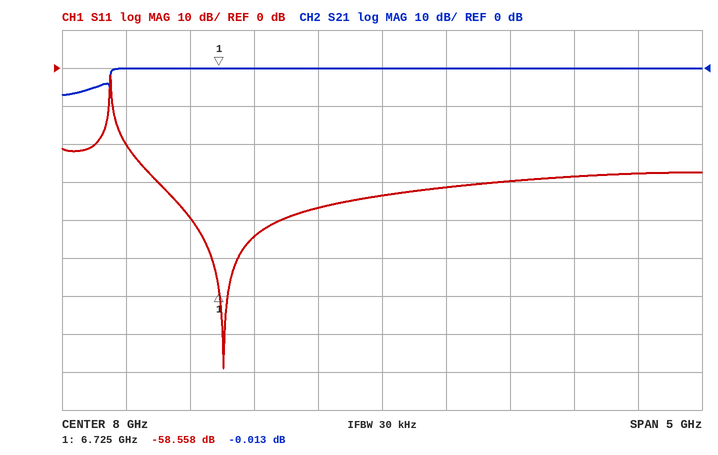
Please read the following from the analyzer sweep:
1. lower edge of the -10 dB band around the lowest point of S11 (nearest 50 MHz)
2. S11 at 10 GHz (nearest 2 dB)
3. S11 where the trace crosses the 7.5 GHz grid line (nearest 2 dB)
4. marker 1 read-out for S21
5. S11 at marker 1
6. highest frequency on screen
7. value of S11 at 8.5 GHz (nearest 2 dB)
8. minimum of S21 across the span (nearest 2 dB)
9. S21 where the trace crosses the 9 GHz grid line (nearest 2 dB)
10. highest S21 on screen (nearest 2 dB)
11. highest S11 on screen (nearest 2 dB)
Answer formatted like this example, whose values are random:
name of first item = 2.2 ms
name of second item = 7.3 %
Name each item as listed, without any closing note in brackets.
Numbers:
lower edge of the -10 dB band around the lowest point of S11 = 5.90 GHz
S11 at 10 GHz = -28 dB
S11 where the trace crosses the 7.5 GHz grid line = -36 dB
marker 1 read-out for S21 = -0.013 dB
S11 at marker 1 = -58.558 dB
highest frequency on screen = 10.5 GHz
value of S11 at 8.5 GHz = -32 dB
minimum of S21 across the span = -8 dB
S21 where the trace crosses the 9 GHz grid line = 0 dB
highest S21 on screen = 0 dB
highest S11 on screen = -2 dB
